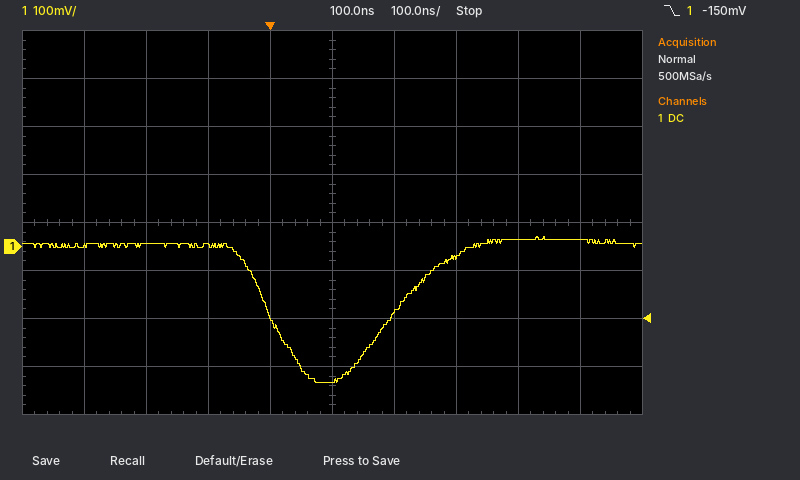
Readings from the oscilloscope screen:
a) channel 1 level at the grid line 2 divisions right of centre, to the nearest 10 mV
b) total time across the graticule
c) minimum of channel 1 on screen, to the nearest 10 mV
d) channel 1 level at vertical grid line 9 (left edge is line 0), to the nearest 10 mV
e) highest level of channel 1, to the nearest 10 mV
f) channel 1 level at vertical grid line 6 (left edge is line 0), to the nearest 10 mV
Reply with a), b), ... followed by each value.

a) -20 mV
b) 1 µs
c) -280 mV
d) 10 mV
e) 20 mV
f) -140 mV
